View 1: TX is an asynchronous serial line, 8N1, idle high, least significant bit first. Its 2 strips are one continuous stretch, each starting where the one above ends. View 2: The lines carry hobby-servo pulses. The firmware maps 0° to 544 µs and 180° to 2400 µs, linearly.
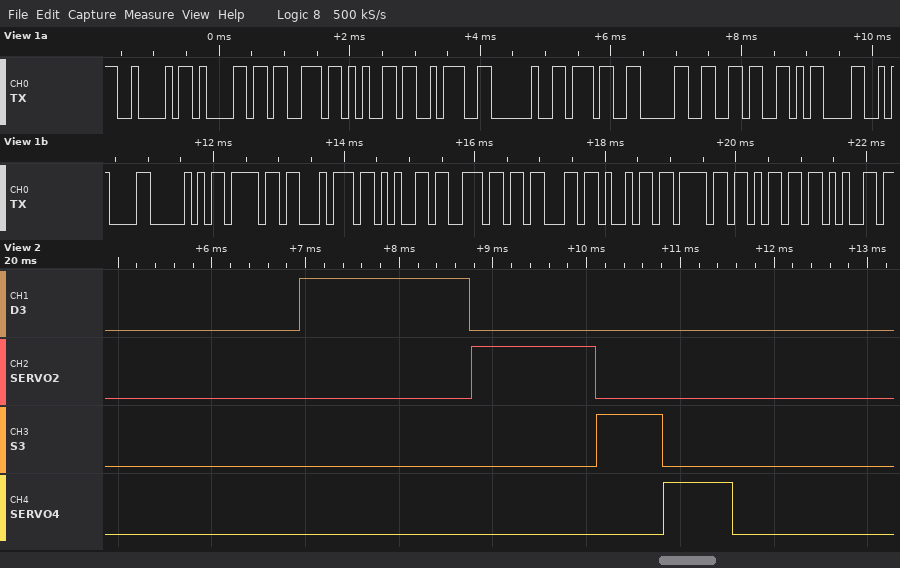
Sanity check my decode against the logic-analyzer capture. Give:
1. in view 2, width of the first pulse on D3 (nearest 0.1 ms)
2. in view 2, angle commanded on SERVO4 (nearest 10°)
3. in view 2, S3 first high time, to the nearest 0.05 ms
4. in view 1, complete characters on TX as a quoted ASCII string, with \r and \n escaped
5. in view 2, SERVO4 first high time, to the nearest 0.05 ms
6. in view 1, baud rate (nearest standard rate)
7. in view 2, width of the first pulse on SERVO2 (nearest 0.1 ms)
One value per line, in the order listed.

1.8 ms
20°
0.70 ms
"Base: 706\r\nPotenciome"
0.75 ms
9600 baud
1.3 ms
